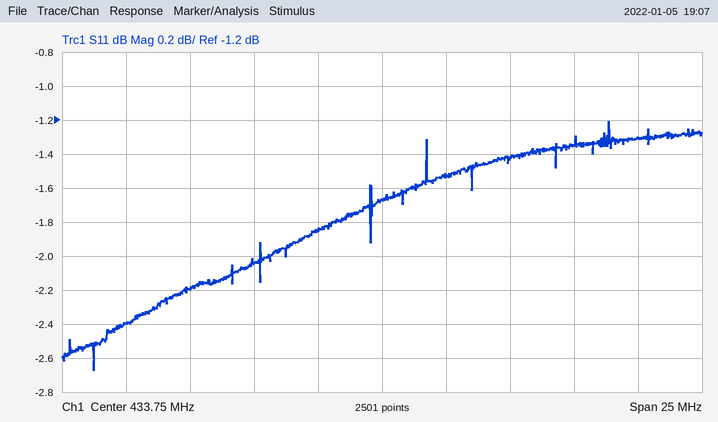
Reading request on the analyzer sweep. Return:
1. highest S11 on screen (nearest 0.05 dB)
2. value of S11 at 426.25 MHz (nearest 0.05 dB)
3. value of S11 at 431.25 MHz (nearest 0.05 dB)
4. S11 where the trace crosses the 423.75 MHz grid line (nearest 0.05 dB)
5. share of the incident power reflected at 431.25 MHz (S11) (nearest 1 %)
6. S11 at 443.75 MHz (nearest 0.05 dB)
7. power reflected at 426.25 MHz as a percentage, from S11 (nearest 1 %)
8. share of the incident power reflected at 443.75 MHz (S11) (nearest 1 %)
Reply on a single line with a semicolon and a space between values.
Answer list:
-1.20 dB; -2.20 dB; -1.85 dB; -2.40 dB; 65 %; -1.30 dB; 60 %; 74 %
